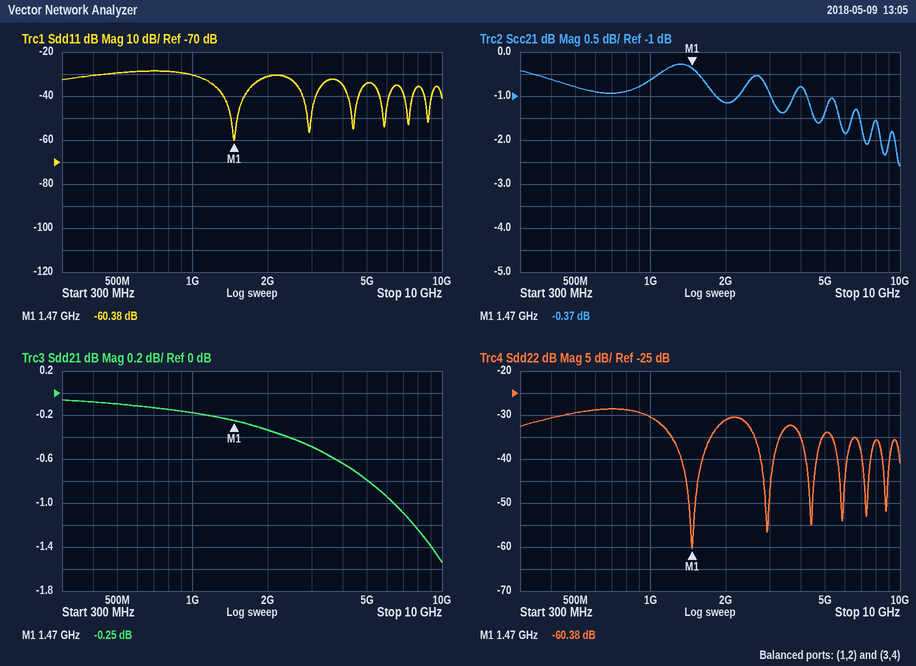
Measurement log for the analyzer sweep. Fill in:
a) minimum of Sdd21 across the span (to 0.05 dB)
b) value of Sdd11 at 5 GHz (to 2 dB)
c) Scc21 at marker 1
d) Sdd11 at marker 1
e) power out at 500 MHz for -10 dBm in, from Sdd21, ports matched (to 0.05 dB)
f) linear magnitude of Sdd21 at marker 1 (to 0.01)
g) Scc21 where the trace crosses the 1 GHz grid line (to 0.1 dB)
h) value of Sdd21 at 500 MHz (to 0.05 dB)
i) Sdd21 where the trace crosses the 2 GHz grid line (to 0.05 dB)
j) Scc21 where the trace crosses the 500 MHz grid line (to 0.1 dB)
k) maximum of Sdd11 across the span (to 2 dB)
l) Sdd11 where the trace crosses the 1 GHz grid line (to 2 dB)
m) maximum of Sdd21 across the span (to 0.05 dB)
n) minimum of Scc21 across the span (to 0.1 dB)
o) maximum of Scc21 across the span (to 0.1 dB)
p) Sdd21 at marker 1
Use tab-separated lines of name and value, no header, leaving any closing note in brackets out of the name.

minimum of Sdd21 across the span	-1.55 dB
value of Sdd11 at 5 GHz	-34 dB
Scc21 at marker 1	-0.37 dB
Sdd11 at marker 1	-60.38 dB
power out at 500 MHz for -10 dBm in, from Sdd21, ports matched	-10.10 dBm
linear magnitude of Sdd21 at marker 1	0.97
Scc21 where the trace crosses the 1 GHz grid line	-0.6 dB
value of Sdd21 at 500 MHz	-0.10 dB
Sdd21 where the trace crosses the 2 GHz grid line	-0.35 dB
Scc21 where the trace crosses the 500 MHz grid line	-0.8 dB
maximum of Sdd11 across the span	-28 dB
Sdd11 where the trace crosses the 1 GHz grid line	-30 dB
maximum of Sdd21 across the span	-0.05 dB
minimum of Scc21 across the span	-2.6 dB
maximum of Scc21 across the span	-0.3 dB
Sdd21 at marker 1	-0.25 dB
